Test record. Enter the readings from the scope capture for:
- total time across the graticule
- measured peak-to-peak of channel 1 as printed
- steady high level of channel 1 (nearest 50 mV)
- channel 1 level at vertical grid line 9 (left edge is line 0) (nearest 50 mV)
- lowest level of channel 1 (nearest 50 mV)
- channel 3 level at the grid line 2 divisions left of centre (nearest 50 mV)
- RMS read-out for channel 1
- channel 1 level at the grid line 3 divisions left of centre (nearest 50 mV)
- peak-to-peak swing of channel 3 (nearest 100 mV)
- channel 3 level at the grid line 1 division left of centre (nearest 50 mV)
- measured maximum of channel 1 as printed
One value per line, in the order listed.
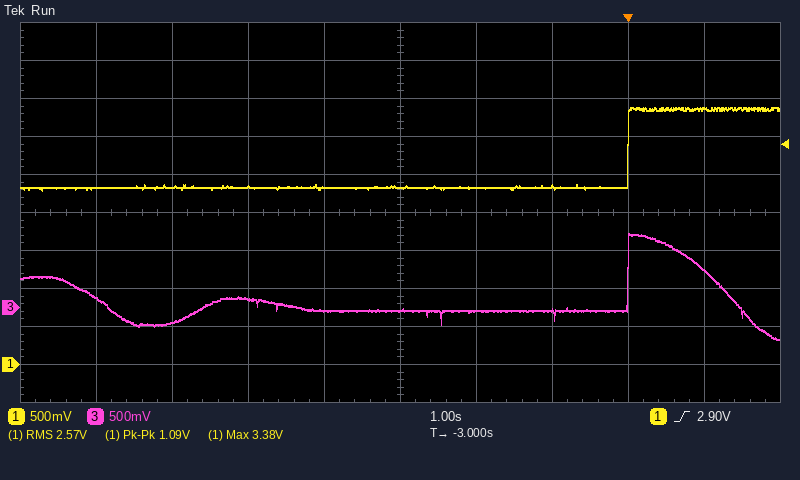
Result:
10 s
1.09 V
3.35 V
3.35 V
2.30 V
100 mV
2.57 V
2.35 V
1.40 V
-50 mV
3.38 V
